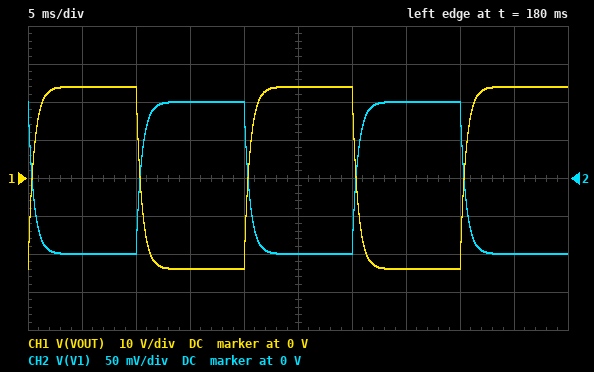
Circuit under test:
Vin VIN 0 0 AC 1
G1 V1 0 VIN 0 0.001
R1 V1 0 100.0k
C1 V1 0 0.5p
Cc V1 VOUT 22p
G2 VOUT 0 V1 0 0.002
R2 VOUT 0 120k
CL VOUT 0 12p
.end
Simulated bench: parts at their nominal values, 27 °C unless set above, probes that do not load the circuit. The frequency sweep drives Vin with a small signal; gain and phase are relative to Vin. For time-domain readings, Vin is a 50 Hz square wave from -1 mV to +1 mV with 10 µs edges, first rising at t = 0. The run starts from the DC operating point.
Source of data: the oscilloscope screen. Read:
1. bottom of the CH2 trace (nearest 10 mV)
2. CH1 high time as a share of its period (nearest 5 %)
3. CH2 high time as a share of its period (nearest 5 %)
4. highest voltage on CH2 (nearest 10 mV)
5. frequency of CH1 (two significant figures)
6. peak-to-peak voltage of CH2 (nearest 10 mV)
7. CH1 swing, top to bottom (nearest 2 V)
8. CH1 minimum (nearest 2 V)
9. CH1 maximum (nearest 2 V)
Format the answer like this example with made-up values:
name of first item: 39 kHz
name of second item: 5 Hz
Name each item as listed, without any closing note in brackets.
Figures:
bottom of the CH2 trace: -100 mV
CH1 high time as a share of its period: 50 %
CH2 high time as a share of its period: 50 %
highest voltage on CH2: 100 mV
frequency of CH1: 50 Hz
peak-to-peak voltage of CH2: 200 mV
CH1 swing, top to bottom: 48 V
CH1 minimum: -24 V
CH1 maximum: 24 V
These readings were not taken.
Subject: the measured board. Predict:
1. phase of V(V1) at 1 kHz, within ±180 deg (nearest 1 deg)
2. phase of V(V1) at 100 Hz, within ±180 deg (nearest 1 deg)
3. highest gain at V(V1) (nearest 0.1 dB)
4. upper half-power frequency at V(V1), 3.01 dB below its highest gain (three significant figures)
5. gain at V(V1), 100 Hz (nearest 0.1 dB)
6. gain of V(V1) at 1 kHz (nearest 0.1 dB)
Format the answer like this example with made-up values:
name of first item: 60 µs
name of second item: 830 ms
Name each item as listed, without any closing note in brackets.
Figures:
phase of V(V1) at 1 kHz, within ±180 deg: 108 deg
phase of V(V1) at 100 Hz, within ±180 deg: 162 deg
highest gain at V(V1): 40.0 dB
upper half-power frequency at V(V1), 3.01 dB below its highest gain: 298 Hz
gain at V(V1), 100 Hz: 39.5 dB
gain of V(V1) at 1 kHz: 29.1 dB
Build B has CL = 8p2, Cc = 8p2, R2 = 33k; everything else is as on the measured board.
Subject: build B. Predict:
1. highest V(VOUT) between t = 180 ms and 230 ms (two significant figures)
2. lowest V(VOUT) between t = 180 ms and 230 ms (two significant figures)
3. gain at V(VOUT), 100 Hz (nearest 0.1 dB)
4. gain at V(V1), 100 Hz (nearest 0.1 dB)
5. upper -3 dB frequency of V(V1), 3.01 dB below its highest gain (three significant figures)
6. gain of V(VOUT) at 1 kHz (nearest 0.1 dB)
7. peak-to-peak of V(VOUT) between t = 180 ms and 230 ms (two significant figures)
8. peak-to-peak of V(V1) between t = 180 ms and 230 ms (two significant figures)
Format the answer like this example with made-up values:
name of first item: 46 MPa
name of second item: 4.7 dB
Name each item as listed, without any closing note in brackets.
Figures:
highest V(VOUT) between t = 180 ms and 230 ms: 6.6 V
lowest V(VOUT) between t = 180 ms and 230 ms: -6.6 V
gain at V(VOUT), 100 Hz: 76.4 dB
gain at V(V1), 100 Hz: 40.0 dB
upper -3 dB frequency of V(V1), 3.01 dB below its highest gain: 2.87 kHz
gain of V(VOUT) at 1 kHz: 75.9 dB
peak-to-peak of V(VOUT) between t = 180 ms and 230 ms: 13 V
peak-to-peak of V(V1) between t = 180 ms and 230 ms: 200 mV
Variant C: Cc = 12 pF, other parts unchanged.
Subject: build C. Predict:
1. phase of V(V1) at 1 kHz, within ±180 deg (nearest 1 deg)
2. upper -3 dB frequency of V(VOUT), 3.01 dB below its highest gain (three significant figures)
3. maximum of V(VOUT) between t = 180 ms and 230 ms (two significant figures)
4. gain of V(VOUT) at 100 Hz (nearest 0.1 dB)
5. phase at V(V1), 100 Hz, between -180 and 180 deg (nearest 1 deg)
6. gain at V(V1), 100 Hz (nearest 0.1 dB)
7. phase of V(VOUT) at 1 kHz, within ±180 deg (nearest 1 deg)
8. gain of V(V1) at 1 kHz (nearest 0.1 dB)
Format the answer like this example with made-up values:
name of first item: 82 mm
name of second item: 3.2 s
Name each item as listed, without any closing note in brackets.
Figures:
phase of V(V1) at 1 kHz, within ±180 deg: 120 deg
upper -3 dB frequency of V(VOUT), 3.01 dB below its highest gain: 545 Hz
maximum of V(VOUT) between t = 180 ms and 230 ms: 24 V
gain of V(VOUT) at 100 Hz: 87.5 dB
phase at V(V1), 100 Hz, between -180 and 180 deg: 170 deg
gain at V(V1), 100 Hz: 39.9 dB
phase of V(VOUT) at 1 kHz, within ±180 deg: -61 deg
gain of V(V1) at 1 kHz: 33.6 dB
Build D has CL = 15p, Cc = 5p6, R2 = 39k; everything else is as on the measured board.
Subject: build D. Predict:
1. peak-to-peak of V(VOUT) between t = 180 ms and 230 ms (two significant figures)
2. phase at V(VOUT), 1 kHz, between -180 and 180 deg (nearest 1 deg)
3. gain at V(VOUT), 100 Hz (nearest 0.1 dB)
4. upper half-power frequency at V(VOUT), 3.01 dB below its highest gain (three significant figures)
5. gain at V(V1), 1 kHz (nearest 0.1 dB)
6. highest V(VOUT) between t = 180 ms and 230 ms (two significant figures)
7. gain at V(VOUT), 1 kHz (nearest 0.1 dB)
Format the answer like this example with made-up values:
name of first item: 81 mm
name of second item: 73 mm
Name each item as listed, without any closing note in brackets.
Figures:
peak-to-peak of V(VOUT) between t = 180 ms and 230 ms: 16 V
phase at V(VOUT), 1 kHz, between -180 and 180 deg: -16 deg
gain at V(VOUT), 100 Hz: 77.8 dB
upper half-power frequency at V(VOUT), 3.01 dB below its highest gain: 3.53 kHz
gain at V(V1), 1 kHz: 39.7 dB
highest V(VOUT) between t = 180 ms and 230 ms: 7.8 V
gain at V(VOUT), 1 kHz: 77.5 dB
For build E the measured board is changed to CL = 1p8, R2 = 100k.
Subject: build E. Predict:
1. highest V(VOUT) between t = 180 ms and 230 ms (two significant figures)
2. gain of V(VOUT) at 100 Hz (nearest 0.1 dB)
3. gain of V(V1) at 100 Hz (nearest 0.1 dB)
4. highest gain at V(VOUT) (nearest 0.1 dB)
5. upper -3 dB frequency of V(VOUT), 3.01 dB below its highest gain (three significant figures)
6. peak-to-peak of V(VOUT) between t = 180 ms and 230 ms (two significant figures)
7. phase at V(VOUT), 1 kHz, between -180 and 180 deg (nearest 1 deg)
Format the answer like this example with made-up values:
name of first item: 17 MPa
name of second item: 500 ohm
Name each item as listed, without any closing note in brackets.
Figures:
highest V(VOUT) between t = 180 ms and 230 ms: 20 V
gain of V(VOUT) at 100 Hz: 85.7 dB
gain of V(V1) at 100 Hz: 39.7 dB
highest gain at V(VOUT): 86.0 dB
upper -3 dB frequency of V(VOUT), 3.01 dB below its highest gain: 358 Hz
peak-to-peak of V(VOUT) between t = 180 ms and 230 ms: 40 V
phase at V(VOUT), 1 kHz, between -180 and 180 deg: -70 deg
